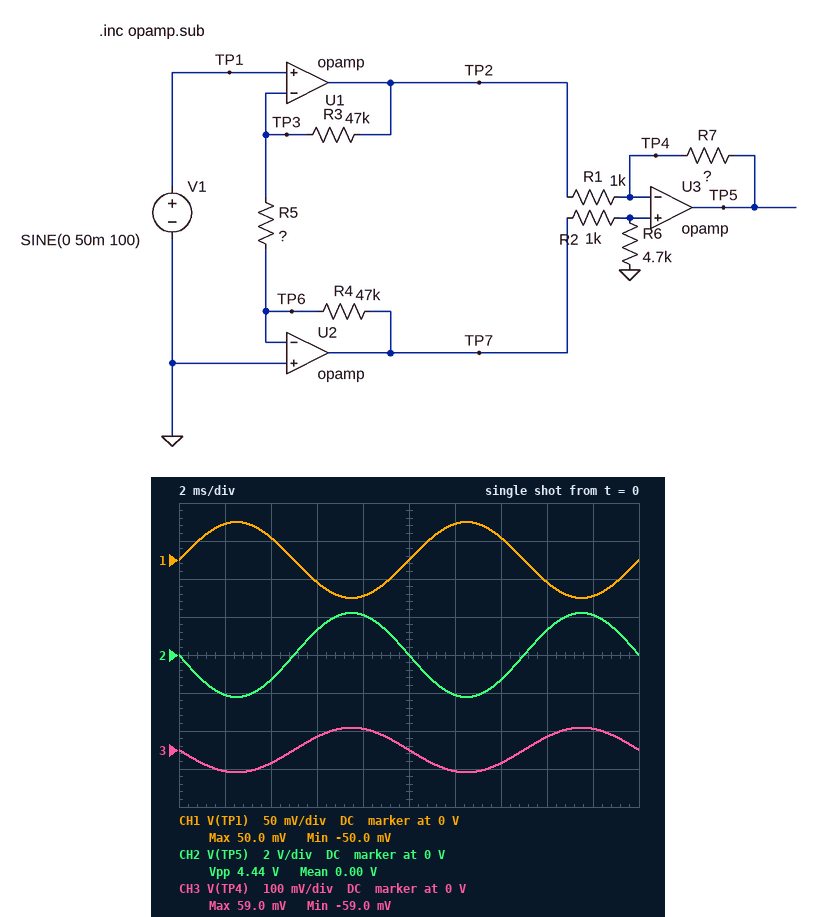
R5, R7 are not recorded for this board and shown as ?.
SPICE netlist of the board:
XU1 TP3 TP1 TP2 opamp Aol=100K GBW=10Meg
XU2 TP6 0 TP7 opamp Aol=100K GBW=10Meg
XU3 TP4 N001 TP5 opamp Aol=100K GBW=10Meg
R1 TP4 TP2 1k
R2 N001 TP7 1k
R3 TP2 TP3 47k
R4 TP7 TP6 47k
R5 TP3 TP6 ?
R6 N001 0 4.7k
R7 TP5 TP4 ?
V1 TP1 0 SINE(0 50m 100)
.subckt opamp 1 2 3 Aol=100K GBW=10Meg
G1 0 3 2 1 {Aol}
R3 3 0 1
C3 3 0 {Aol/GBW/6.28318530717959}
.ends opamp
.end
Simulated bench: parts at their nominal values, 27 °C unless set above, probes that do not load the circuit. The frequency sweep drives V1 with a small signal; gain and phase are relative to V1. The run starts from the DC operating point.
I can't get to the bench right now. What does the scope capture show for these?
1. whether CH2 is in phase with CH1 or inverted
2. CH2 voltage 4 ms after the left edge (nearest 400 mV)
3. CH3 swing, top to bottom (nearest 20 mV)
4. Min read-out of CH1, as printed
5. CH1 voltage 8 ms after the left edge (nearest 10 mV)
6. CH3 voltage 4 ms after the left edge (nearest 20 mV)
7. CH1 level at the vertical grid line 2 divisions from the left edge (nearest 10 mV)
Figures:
inverted
-1.2 V
120 mV
-50.0 mV
-50 mV
-40 mV
30 mV
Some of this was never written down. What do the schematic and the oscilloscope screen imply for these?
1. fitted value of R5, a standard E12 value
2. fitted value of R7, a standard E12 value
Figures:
33 kΩ
12 kΩ
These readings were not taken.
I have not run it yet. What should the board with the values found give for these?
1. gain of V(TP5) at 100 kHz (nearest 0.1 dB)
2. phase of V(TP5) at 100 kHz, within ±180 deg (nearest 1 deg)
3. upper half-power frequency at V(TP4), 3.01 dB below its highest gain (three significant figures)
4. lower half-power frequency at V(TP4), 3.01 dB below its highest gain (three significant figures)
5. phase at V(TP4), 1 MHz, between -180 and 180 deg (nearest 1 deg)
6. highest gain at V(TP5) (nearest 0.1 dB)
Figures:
32.9 dB
170 deg
4.11 MHz
277 kHz
40 deg
32.9 dB
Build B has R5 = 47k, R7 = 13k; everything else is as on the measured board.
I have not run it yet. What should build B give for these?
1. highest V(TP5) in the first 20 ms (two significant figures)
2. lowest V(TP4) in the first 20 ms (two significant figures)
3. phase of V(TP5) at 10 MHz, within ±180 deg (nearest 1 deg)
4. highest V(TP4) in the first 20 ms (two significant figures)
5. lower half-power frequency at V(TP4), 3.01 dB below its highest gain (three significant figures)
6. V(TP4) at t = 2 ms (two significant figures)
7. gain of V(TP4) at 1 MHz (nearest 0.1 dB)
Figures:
1.9 V
-41 mV
24 deg
41 mV
386 kHz
-39 mV
4.0 dB
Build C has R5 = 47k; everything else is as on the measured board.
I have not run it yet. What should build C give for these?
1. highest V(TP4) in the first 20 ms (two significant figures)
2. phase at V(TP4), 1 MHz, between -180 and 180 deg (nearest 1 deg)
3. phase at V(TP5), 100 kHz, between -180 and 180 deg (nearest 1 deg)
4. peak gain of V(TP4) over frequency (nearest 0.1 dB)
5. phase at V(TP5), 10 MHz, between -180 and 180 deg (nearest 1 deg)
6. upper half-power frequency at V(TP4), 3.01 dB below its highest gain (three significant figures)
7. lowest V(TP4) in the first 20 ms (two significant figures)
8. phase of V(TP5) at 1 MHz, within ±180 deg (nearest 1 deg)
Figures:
41 mV
41 deg
171 deg
4.2 dB
24 deg
5.16 MHz
-41 mV
111 deg
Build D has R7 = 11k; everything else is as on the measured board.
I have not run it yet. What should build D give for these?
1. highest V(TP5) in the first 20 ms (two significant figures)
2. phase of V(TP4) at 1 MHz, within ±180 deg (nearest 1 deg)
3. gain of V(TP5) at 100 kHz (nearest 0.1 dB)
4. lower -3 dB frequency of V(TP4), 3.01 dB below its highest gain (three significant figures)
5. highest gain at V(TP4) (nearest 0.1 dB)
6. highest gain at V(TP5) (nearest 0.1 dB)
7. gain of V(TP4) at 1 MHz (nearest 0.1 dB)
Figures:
2.0 V
44 deg
32.1 dB
279 kHz
5.5 dB
32.2 dB
5.3 dB
